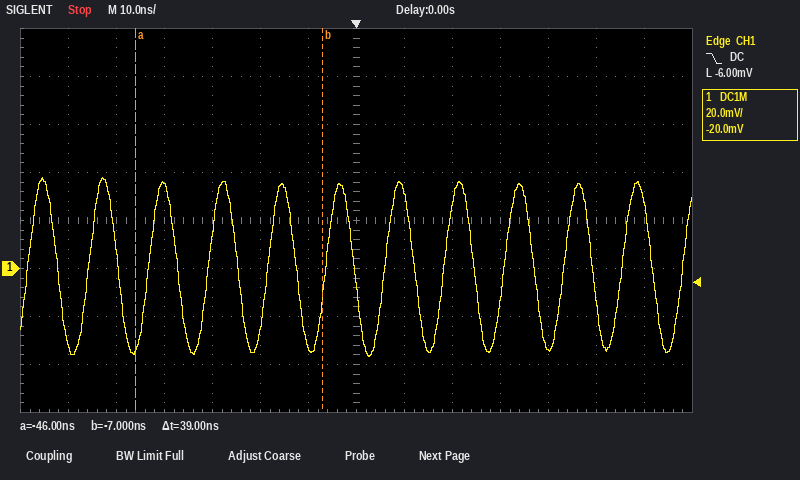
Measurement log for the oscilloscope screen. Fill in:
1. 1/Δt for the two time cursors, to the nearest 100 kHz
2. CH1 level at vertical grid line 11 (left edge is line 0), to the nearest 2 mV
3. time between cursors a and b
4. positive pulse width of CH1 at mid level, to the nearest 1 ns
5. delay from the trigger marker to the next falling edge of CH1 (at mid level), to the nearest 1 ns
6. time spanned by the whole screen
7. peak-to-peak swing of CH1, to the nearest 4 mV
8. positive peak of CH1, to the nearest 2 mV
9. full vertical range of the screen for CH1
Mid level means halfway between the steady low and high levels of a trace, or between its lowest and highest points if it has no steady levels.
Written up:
25.6 MHz
-34 mV
39 ns
6 ns
12 ns
140 ns
76 mV
38 mV
160 mV
